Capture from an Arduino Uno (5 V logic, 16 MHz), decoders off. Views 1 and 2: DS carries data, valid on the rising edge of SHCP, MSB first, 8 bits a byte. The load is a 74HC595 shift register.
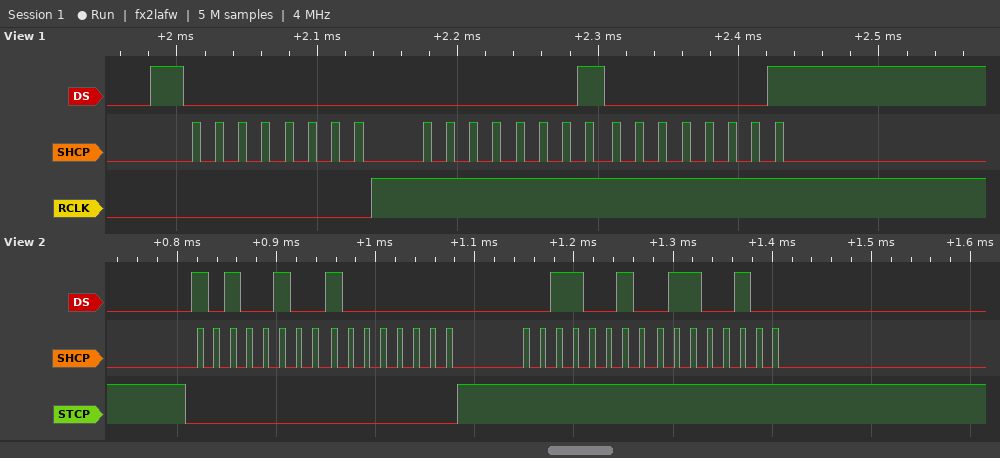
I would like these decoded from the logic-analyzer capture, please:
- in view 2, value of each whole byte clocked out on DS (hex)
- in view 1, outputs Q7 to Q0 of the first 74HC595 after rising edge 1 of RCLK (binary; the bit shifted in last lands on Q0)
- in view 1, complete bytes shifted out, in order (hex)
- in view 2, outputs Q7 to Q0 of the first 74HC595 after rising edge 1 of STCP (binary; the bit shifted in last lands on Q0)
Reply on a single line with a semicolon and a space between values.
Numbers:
A4 80 32 64; 00000000; 0x00 0x01 0x01; 10000000
